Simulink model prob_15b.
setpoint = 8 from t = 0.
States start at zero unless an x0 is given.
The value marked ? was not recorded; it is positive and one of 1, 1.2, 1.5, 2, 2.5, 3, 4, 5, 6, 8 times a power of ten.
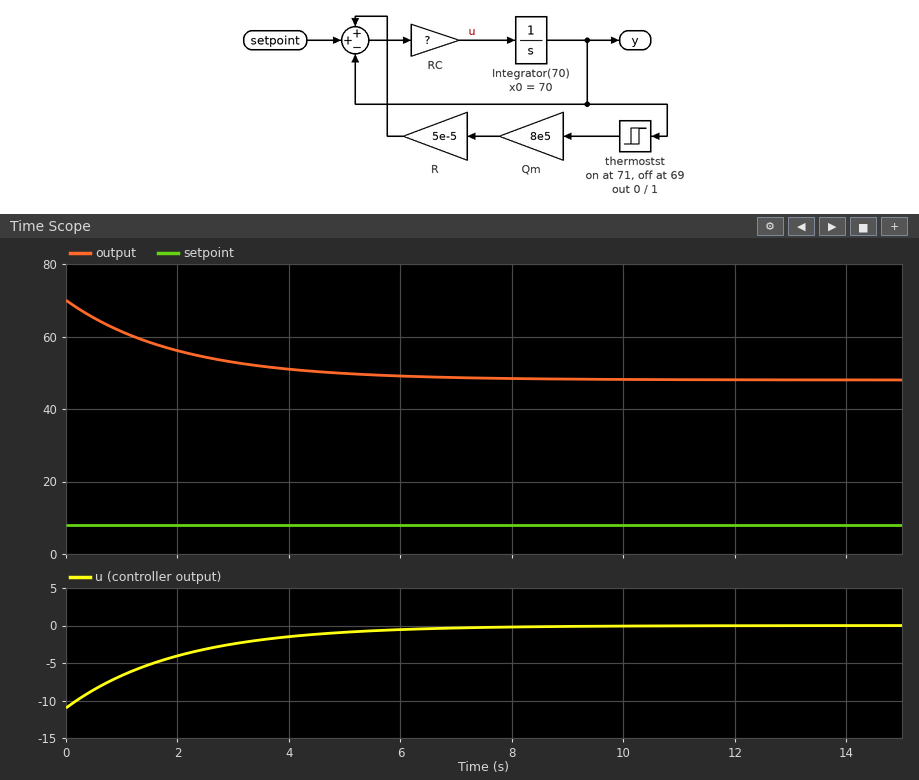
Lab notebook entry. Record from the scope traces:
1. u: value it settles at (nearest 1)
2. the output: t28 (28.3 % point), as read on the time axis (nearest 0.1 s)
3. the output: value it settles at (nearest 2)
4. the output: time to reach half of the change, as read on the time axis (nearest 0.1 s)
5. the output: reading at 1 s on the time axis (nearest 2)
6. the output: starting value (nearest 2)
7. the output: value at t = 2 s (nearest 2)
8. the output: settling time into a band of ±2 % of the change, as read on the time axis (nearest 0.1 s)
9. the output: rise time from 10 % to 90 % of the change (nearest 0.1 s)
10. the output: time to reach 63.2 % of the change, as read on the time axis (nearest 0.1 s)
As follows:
0
0.7 s
48
1.4 s
62
70
56
7.8 s
4.4 s
2.0 s
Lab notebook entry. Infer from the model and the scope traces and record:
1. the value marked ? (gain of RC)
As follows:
0.5
